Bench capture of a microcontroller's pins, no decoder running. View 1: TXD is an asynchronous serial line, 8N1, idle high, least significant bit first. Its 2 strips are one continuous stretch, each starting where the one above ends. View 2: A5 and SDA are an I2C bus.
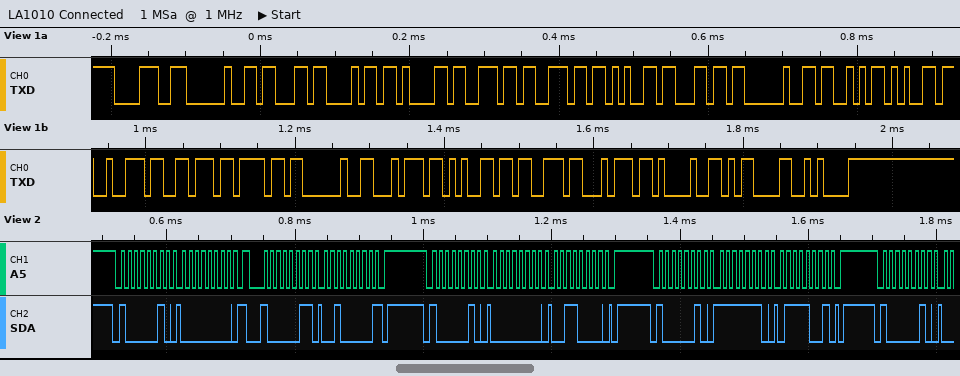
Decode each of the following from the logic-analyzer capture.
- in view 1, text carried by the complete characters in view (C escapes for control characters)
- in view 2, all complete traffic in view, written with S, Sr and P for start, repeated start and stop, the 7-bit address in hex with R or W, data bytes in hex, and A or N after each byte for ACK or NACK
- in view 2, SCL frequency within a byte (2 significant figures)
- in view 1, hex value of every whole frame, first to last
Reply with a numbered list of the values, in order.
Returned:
1. "8 channel Servo test!\r\n"
2. S 41W A 00 A Sr 41R A 20 N P S 41W A 00 A 30 A P S 41W A FE A 79 A P S 41W A
3. 100 kHz
4. 38 20 63 68 61 6E 6E 65 6C 20 53 65 72 76 6F 20 74 65 73 74 21 0D 0A
